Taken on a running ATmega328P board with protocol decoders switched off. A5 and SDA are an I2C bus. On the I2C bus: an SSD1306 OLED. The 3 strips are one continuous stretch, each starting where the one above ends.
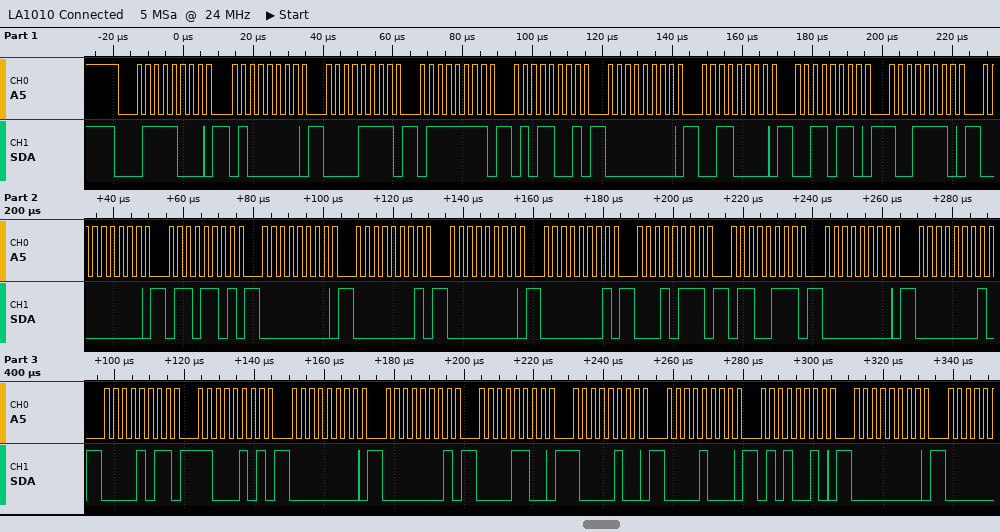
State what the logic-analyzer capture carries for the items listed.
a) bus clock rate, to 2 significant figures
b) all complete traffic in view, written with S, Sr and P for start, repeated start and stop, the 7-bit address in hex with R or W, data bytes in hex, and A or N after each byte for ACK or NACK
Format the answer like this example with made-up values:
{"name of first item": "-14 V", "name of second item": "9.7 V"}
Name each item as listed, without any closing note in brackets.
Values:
{"bus clock rate, to 2 significant figures": "400 kHz", "all complete traffic in view, written with S, Sr and P for start, repeated start and stop, the 7-bit address in hex with R or W, data bytes in hex, and A or N after each byte for ACK or NACK": "S 3CW A 40 A 0F A 7F A 59 A 00 A 30 A 36 A 9E A 00 A 6D A 00 A 01 A 00 A 01 A 17 A 67 A 00 A 01 A 0B A C5 A 00 A 01 A 0C A 84 A 08 A 52 A 00 A"}
